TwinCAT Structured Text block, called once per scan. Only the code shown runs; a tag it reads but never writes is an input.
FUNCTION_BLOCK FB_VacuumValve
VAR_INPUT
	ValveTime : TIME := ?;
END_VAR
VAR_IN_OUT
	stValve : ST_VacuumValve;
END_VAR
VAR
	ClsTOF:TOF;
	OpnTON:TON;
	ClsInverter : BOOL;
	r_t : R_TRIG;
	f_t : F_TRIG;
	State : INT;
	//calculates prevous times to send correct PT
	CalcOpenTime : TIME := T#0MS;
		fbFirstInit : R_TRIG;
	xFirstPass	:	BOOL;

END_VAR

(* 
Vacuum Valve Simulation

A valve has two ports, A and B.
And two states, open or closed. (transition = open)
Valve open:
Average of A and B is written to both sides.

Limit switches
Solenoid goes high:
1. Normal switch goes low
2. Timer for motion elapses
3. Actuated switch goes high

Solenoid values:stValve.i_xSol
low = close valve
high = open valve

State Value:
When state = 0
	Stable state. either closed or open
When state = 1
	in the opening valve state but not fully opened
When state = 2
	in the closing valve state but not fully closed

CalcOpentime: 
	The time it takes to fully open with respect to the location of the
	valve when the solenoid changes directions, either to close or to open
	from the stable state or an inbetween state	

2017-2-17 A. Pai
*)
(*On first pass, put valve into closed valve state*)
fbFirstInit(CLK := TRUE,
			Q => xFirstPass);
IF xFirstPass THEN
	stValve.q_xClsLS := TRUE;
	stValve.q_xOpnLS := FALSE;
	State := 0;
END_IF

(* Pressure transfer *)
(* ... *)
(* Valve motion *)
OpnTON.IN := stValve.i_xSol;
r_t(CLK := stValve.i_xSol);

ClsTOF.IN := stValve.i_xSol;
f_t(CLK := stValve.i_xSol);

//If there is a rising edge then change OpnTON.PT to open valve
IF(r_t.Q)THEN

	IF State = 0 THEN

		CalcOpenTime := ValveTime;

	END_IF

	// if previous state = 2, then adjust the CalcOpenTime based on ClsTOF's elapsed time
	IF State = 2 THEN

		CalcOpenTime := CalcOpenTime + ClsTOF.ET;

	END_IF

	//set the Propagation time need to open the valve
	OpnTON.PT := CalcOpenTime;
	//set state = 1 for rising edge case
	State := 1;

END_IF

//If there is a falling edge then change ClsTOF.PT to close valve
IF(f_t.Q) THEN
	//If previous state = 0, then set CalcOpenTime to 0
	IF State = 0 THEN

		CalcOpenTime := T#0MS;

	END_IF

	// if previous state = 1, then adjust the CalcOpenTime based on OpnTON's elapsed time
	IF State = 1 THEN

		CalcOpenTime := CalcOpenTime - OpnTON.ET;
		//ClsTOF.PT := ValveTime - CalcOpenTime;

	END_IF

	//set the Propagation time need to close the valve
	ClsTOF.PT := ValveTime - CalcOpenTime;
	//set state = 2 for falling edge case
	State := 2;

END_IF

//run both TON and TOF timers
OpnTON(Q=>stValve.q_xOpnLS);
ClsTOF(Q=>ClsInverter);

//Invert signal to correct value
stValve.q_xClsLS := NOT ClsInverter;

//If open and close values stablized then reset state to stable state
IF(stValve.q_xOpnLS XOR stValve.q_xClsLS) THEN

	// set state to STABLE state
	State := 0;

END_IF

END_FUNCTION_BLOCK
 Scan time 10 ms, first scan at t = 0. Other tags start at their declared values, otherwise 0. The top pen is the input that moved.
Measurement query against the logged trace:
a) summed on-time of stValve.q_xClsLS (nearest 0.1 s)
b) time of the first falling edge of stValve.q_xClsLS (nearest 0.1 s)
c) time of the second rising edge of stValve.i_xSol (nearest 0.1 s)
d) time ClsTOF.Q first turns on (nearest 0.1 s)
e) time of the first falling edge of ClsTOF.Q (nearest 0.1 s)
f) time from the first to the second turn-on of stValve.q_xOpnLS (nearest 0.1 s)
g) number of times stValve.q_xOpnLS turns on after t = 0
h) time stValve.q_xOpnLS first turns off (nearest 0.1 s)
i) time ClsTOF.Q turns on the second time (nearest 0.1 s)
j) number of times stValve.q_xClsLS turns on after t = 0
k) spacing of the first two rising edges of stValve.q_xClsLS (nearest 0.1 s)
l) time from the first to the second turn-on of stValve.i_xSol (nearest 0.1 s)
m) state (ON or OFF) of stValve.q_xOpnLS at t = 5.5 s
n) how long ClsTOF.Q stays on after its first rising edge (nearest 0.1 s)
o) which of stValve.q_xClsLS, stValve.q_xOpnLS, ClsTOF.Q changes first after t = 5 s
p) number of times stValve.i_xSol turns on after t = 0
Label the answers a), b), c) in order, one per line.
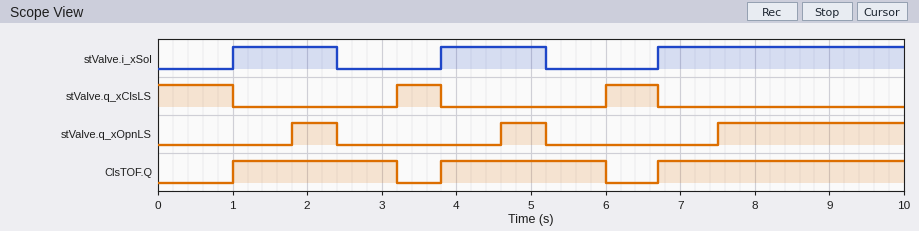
a) 2.3 s
b) 1.0 s
c) 3.8 s
d) 1.0 s
e) 3.2 s
f) 2.8 s
g) 3
h) 2.4 s
i) 3.8 s
j) 2
k) 2.8 s
l) 2.8 s
m) OFF
n) 2.2 s
o) stValve.q_xOpnLS
p) 3
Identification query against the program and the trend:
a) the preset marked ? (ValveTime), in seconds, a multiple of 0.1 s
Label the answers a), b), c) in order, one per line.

a) 0.8 s
